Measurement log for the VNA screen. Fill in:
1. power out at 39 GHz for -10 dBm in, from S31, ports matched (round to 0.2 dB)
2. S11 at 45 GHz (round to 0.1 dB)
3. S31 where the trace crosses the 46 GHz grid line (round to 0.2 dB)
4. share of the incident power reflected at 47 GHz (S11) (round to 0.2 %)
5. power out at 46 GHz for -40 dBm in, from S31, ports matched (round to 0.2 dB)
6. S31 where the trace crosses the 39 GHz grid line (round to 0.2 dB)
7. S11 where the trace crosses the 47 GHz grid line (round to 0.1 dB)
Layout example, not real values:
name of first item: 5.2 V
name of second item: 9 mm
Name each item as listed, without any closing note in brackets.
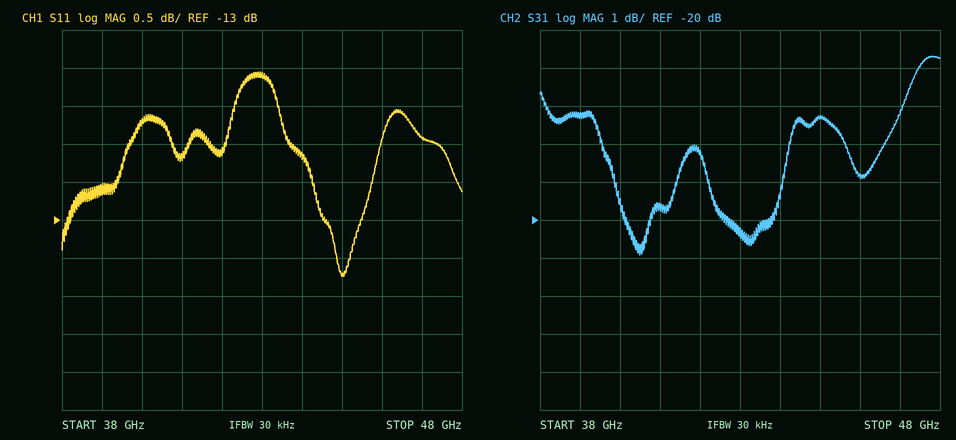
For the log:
power out at 39 GHz for -10 dBm in, from S31, ports matched: -27.2 dBm
S11 at 45 GHz: -13.7 dB
S31 where the trace crosses the 46 GHz grid line: -18.8 dB
share of the incident power reflected at 47 GHz (S11): 6.4 %
power out at 46 GHz for -40 dBm in, from S31, ports matched: -58.8 dBm
S31 where the trace crosses the 39 GHz grid line: -17.2 dB
S11 where the trace crosses the 47 GHz grid line: -11.9 dB
